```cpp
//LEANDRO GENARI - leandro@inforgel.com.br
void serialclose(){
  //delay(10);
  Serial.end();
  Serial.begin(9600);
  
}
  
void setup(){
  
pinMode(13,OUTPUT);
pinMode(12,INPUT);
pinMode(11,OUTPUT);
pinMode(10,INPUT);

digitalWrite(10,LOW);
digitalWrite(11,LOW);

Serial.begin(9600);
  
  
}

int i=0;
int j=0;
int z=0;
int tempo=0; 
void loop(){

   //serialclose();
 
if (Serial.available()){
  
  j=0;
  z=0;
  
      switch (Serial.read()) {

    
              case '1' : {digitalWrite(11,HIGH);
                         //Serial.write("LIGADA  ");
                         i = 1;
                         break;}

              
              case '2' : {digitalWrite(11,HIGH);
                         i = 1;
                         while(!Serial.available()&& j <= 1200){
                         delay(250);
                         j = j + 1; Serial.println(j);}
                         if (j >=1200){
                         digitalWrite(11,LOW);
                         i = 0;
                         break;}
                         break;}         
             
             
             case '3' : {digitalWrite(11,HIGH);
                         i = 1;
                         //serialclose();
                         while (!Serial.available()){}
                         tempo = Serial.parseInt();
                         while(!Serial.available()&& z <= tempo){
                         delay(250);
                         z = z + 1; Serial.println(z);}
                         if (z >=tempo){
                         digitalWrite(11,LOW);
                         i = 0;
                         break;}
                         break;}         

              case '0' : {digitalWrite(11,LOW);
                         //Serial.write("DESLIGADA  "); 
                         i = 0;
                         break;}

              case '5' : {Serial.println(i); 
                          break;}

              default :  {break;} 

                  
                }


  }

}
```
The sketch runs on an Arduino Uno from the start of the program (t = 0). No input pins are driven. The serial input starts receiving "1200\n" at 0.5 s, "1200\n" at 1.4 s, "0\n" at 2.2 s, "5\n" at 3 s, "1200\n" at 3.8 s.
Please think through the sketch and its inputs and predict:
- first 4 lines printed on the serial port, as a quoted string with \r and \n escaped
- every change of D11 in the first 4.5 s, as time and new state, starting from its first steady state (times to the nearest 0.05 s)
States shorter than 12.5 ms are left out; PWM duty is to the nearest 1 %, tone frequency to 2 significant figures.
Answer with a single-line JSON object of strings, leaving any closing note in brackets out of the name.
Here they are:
{"first 4 lines printed on the serial port, as a quoted string with \\r and \\n escaped": "\"1\\r\\n1\\r\\n0\\r\\n1\\r\\n\"", "every change of D11 in the first 4.5 s, as time and new state, starting from its first steady state": "0 s low; 0.5 s high; 0.75 s low; 1.4 s high; 1.65 s low; 3.8 s high; 4.05 s low"}
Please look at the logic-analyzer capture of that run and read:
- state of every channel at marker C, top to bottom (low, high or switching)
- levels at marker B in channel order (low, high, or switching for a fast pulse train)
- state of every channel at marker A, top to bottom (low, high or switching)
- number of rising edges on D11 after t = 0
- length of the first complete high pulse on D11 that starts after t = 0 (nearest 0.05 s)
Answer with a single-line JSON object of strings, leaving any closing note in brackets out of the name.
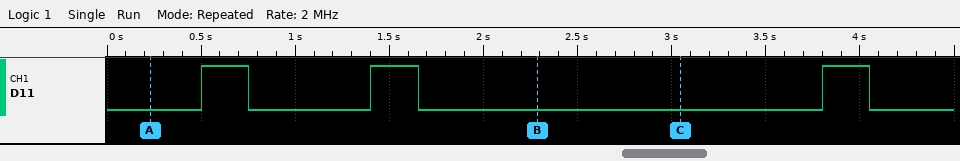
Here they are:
{"state of every channel at marker C, top to bottom": "D11 low", "levels at marker B in channel order": "D11 low", "state of every channel at marker A, top to bottom": "D11 low", "number of rising edges on D11 after t = 0": "3", "length of the first complete high pulse on D11 that starts after t = 0": "0.25 s"}
